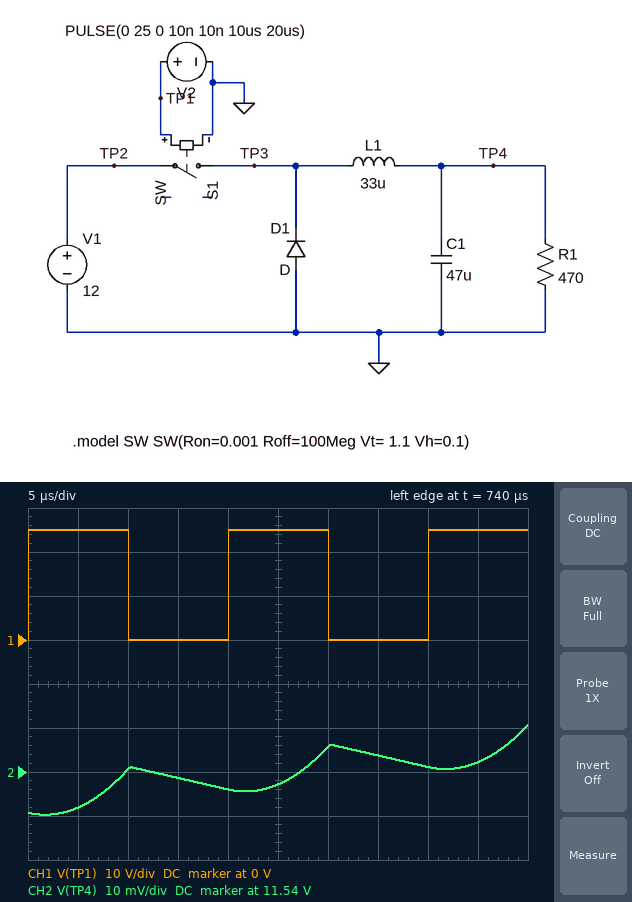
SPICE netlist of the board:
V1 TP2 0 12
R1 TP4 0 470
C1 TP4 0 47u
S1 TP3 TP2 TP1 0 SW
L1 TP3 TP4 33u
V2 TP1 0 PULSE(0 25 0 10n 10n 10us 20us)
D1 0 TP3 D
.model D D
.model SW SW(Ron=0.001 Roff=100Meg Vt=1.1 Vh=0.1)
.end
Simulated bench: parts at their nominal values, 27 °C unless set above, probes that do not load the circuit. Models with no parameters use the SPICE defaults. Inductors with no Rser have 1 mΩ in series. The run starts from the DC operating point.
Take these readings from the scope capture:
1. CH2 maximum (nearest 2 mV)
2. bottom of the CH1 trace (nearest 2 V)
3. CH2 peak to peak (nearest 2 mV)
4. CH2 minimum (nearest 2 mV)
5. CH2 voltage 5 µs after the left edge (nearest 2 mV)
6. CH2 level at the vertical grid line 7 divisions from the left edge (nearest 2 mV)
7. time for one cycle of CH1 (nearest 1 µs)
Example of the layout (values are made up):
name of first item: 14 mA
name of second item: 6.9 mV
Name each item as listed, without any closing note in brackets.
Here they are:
CH2 maximum: 11.550 V
bottom of the CH1 trace: 0 V
CH2 peak to peak: 20 mV
CH2 minimum: 11.530 V
CH2 voltage 5 µs after the left edge: 11.532 V
CH2 level at the vertical grid line 7 divisions from the left edge: 11.544 V
time for one cycle of CH1: 20 µs
